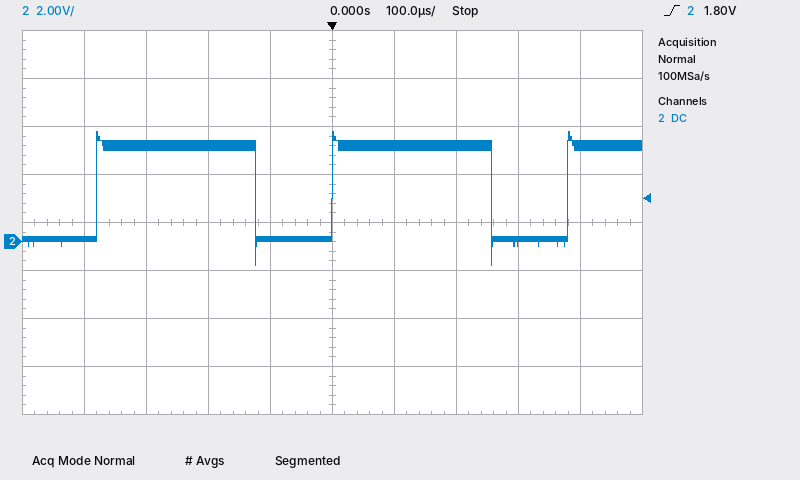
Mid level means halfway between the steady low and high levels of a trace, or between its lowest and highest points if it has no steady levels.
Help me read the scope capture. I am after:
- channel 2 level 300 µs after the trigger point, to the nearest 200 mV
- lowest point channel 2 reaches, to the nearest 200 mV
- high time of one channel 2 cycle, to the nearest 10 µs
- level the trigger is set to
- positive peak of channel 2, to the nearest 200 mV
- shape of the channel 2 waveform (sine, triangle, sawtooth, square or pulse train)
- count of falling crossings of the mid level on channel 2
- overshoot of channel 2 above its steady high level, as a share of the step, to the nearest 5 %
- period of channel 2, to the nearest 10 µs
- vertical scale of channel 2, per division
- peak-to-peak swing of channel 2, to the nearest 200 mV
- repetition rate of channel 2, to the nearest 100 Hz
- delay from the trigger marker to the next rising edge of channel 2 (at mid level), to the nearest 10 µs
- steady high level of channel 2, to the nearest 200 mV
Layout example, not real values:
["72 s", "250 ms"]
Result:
["0.0 V", "-1.0 V", "260 µs", "1.80 V", "4.6 V", "pulse train", "2", "15 %", "380 µs", "2 V", "5.6 V", "2.6 kHz", "380 µs", "4.0 V"]
